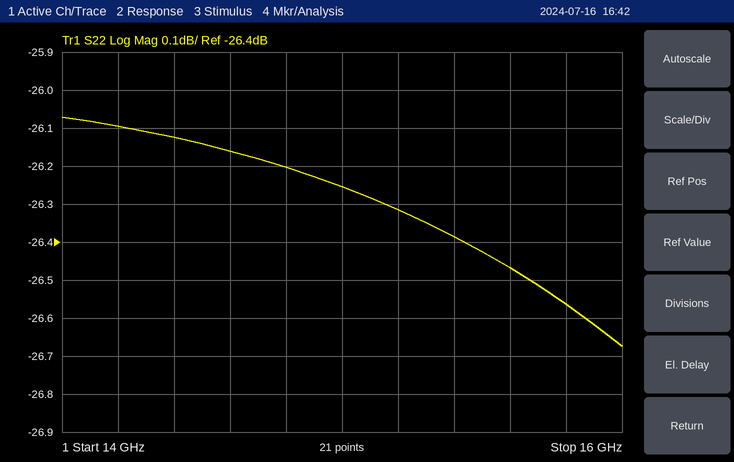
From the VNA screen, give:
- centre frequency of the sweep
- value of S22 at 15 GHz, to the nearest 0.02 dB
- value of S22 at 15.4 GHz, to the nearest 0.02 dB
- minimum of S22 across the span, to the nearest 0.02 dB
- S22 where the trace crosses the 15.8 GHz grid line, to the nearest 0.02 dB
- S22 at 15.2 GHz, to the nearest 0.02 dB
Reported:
15 GHz
-26.26 dB
-26.38 dB
-26.68 dB
-26.56 dB
-26.32 dB
